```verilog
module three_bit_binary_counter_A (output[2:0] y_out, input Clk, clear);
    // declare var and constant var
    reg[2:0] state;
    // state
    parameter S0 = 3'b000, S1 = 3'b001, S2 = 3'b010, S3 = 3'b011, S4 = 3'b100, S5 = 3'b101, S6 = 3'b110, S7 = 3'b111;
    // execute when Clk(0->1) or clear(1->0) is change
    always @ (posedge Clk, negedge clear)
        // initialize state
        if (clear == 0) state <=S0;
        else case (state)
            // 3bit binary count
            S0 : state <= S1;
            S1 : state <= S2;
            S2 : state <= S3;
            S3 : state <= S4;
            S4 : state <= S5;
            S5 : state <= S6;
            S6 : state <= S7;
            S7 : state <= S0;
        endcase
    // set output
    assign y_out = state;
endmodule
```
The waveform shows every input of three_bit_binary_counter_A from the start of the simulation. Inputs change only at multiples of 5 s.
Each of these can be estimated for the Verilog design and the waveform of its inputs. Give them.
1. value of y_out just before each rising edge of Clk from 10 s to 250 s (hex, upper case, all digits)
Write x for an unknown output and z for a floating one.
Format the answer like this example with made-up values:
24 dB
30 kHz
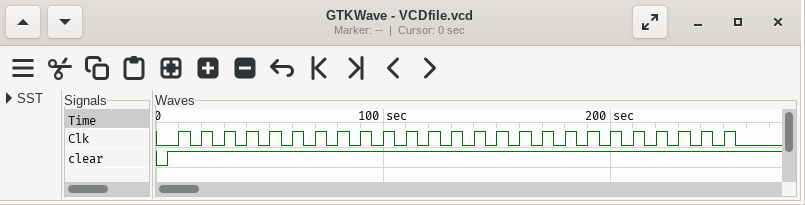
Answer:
0, 1, 2, 3, 4, 5, 6, 7, 0, 1, 2, 3, 4, 5, 6, 7, 0, 1, 2, 3, 4, 5, 6, 7, 0
